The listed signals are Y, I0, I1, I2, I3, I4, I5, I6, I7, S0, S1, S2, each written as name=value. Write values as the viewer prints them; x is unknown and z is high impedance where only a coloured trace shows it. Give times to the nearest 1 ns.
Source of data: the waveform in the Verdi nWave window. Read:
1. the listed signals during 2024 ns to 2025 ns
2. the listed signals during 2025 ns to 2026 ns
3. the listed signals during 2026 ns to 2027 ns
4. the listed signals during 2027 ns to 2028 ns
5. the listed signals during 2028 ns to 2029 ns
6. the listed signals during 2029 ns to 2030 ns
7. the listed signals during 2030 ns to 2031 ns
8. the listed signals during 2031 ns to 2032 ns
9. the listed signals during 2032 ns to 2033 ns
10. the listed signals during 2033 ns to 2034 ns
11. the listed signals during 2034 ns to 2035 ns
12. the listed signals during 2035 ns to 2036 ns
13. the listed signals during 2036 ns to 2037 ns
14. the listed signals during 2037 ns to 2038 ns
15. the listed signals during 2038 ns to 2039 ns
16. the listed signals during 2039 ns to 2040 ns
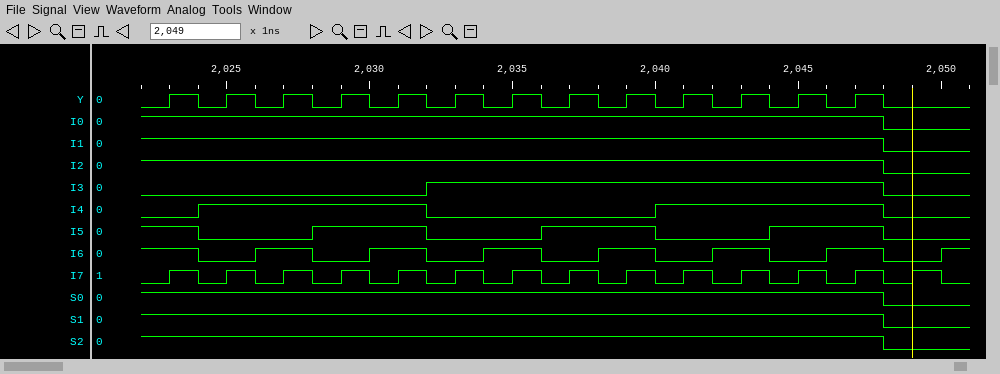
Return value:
Y=0, I0=1, I1=1, I2=1, I3=0, I4=1, I5=0, I6=0, I7=0, S0=1, S1=1, S2=1
Y=1, I0=1, I1=1, I2=1, I3=0, I4=1, I5=0, I6=0, I7=1, S0=1, S1=1, S2=1
Y=0, I0=1, I1=1, I2=1, I3=0, I4=1, I5=0, I6=1, I7=0, S0=1, S1=1, S2=1
Y=1, I0=1, I1=1, I2=1, I3=0, I4=1, I5=0, I6=1, I7=1, S0=1, S1=1, S2=1
Y=0, I0=1, I1=1, I2=1, I3=0, I4=1, I5=1, I6=0, I7=0, S0=1, S1=1, S2=1
Y=1, I0=1, I1=1, I2=1, I3=0, I4=1, I5=1, I6=0, I7=1, S0=1, S1=1, S2=1
Y=0, I0=1, I1=1, I2=1, I3=0, I4=1, I5=1, I6=1, I7=0, S0=1, S1=1, S2=1
Y=1, I0=1, I1=1, I2=1, I3=0, I4=1, I5=1, I6=1, I7=1, S0=1, S1=1, S2=1
Y=0, I0=1, I1=1, I2=1, I3=1, I4=0, I5=0, I6=0, I7=0, S0=1, S1=1, S2=1
Y=1, I0=1, I1=1, I2=1, I3=1, I4=0, I5=0, I6=0, I7=1, S0=1, S1=1, S2=1
Y=0, I0=1, I1=1, I2=1, I3=1, I4=0, I5=0, I6=1, I7=0, S0=1, S1=1, S2=1
Y=1, I0=1, I1=1, I2=1, I3=1, I4=0, I5=0, I6=1, I7=1, S0=1, S1=1, S2=1
Y=0, I0=1, I1=1, I2=1, I3=1, I4=0, I5=1, I6=0, I7=0, S0=1, S1=1, S2=1
Y=1, I0=1, I1=1, I2=1, I3=1, I4=0, I5=1, I6=0, I7=1, S0=1, S1=1, S2=1
Y=0, I0=1, I1=1, I2=1, I3=1, I4=0, I5=1, I6=1, I7=0, S0=1, S1=1, S2=1
Y=1, I0=1, I1=1, I2=1, I3=1, I4=0, I5=1, I6=1, I7=1, S0=1, S1=1, S2=1
